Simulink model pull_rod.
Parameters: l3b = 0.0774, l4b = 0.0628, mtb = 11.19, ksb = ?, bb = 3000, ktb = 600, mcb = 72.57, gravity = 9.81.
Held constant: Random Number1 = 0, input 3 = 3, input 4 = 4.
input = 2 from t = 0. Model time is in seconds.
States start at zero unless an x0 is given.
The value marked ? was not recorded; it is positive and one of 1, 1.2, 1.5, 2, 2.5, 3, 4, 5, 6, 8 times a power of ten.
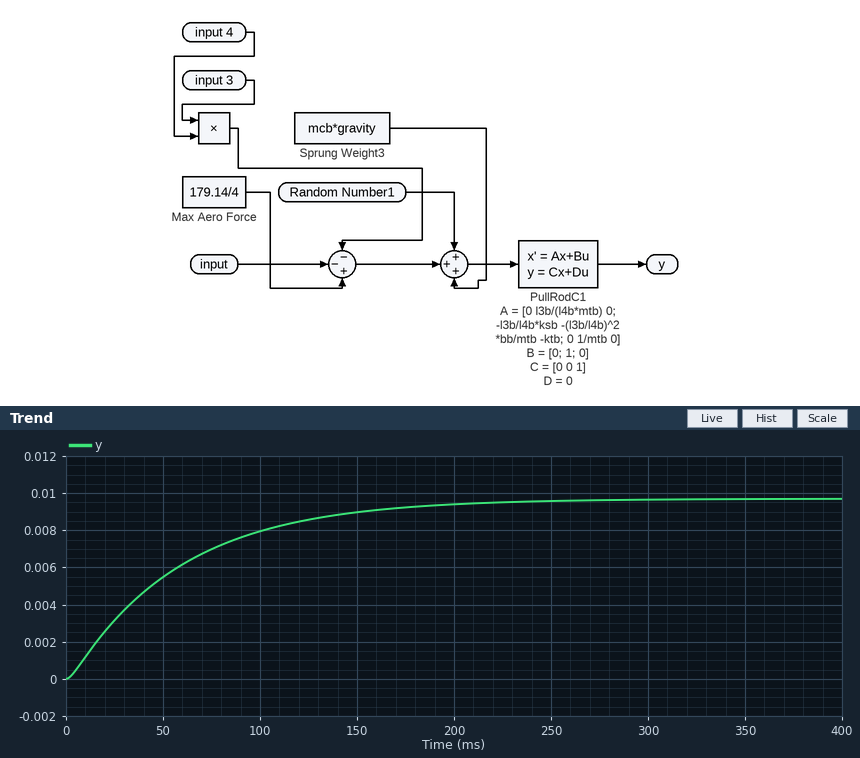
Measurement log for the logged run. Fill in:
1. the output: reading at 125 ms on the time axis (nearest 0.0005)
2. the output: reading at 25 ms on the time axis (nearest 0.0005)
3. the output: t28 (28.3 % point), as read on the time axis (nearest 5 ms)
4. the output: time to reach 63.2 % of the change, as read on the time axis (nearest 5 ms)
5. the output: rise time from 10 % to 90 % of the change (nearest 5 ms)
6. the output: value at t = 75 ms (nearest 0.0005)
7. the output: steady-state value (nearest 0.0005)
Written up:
0.0085
0.0030
20 ms
60 ms
125 ms
0.0070
0.0095
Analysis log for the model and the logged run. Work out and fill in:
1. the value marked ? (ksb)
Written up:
50000
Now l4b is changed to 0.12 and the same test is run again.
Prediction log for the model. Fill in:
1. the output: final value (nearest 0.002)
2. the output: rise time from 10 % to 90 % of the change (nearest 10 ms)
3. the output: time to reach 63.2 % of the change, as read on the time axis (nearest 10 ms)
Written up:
0.034
110 ms
60 ms
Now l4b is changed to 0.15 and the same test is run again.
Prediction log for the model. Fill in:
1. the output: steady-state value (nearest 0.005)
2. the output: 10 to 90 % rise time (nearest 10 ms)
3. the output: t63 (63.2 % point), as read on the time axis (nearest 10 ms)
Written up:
0.055
100 ms
60 ms
